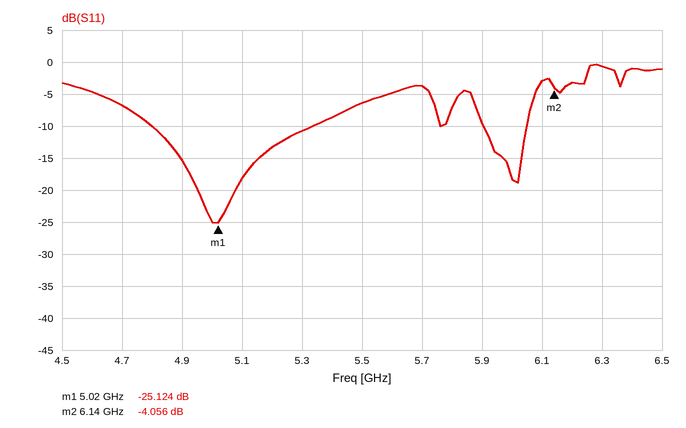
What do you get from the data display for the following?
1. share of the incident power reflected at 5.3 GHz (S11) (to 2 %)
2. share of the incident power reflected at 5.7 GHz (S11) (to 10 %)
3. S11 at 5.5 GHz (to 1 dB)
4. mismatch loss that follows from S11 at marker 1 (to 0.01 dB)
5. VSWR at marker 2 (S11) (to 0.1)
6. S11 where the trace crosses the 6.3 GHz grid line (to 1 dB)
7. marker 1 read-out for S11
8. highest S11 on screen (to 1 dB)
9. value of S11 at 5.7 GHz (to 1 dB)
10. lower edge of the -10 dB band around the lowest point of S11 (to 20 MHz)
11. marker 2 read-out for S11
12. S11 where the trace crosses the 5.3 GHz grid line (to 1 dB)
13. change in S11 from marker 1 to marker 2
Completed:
8 %
40 %
-6 dB
0.01 dB
4.4
-1 dB
-25.124 dB
0 dB
-4 dB
4.80 GHz
-4.056 dB
-11 dB
21.068 dB
